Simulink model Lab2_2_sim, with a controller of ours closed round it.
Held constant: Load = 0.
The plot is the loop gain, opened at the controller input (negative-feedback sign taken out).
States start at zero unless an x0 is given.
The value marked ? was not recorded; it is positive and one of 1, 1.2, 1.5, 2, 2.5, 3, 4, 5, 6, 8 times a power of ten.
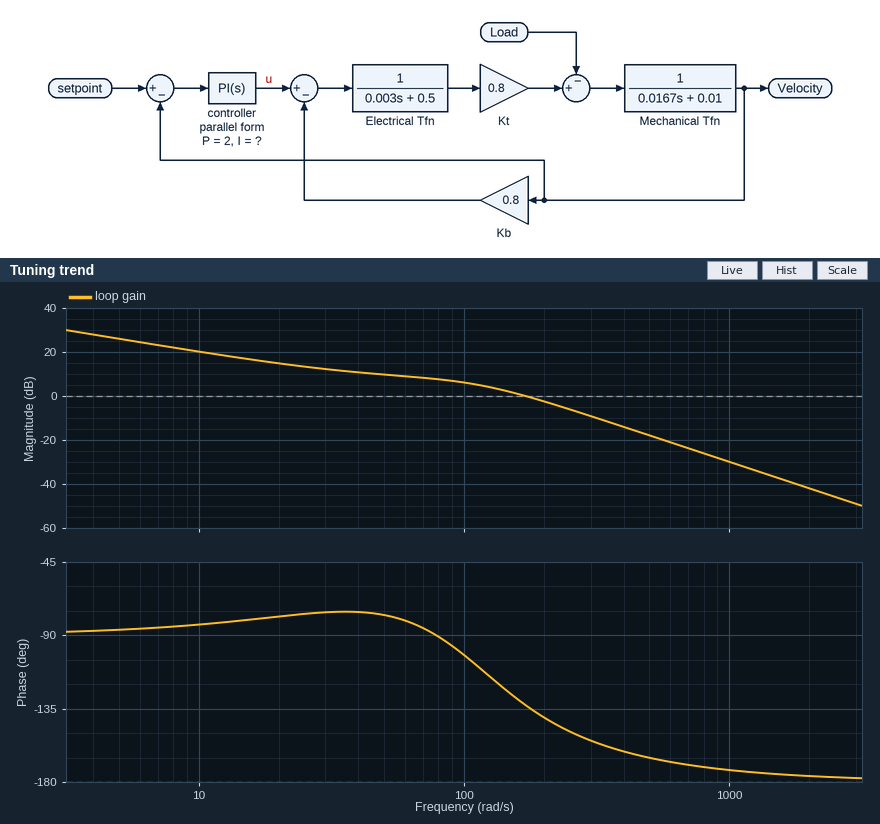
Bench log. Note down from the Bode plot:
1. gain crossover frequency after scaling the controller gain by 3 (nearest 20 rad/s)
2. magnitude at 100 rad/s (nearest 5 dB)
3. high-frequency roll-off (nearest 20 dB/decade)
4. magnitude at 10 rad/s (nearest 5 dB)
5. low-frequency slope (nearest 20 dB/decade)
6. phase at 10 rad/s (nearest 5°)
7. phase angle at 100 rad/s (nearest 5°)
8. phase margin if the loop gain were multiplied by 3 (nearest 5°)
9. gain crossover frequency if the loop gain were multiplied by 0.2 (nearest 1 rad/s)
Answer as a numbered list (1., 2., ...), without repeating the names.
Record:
1. 300 rad/s
2. 5 dB
3. -40 dB/decade
4. 20 dB
5. -20 dB/decade
6. -85°
7. -100°
8. 25°
9. 23 rad/s
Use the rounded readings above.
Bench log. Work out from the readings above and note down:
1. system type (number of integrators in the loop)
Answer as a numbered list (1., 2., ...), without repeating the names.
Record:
1. 1
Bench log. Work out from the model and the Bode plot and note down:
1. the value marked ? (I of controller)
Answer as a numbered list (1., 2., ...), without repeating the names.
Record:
1. 80
